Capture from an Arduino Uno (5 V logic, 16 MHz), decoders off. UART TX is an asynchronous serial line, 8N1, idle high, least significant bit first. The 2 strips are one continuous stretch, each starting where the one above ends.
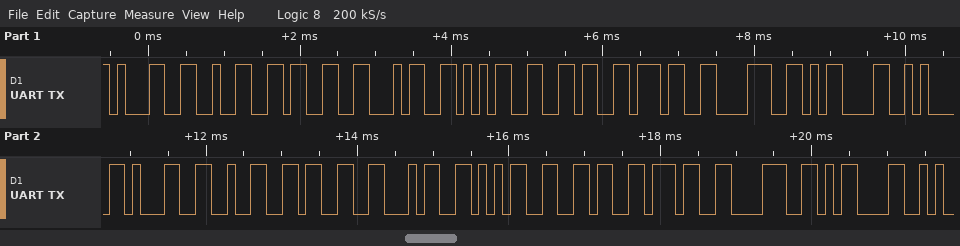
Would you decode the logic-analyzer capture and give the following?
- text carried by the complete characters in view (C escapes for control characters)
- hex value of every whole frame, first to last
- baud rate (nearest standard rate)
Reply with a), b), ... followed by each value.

a) "12345678\r\n12345678\r"
b) 0x31 0x32 0x33 0x34 0x35 0x36 0x37 0x38 0x0D 0x0A 0x31 0x32 0x33 0x34 0x35 0x36 0x37 0x38 0x0D
c) 9600 baud
